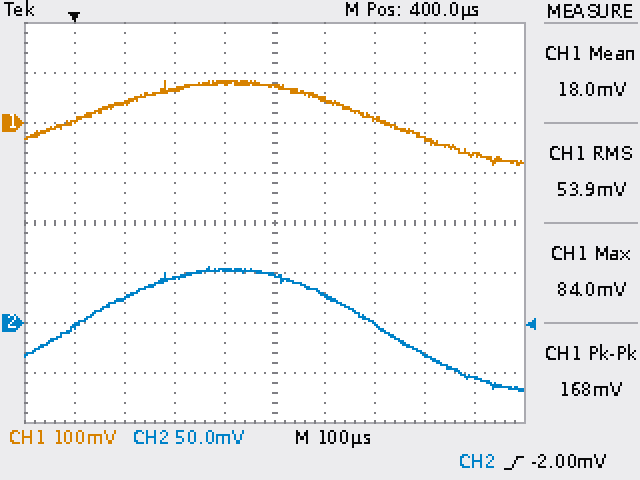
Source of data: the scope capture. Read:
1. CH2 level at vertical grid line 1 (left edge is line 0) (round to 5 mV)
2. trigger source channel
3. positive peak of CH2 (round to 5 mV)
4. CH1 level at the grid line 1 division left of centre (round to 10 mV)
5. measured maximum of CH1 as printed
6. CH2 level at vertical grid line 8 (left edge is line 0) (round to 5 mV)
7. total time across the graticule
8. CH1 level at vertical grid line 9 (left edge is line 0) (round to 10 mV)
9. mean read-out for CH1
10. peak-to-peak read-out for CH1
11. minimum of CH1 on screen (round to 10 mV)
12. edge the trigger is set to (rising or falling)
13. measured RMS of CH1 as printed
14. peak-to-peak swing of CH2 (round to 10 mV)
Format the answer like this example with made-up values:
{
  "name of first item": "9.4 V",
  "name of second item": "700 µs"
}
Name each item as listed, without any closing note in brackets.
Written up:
{
  "CH2 level at vertical grid line 1 (left edge is line 0)": "-5 mV",
  "trigger source channel": "CH2",
  "positive peak of CH2": "55 mV",
  "CH1 level at the grid line 1 division left of centre": "80 mV",
  "measured maximum of CH1 as printed": "84.0 mV",
  "CH2 level at vertical grid line 8 (left edge is line 0)": "-30 mV",
  "total time across the graticule": "1 ms",
  "CH1 level at vertical grid line 9 (left edge is line 0)": "-60 mV",
  "mean read-out for CH1": "18.0 mV",
  "peak-to-peak read-out for CH1": "168 mV",
  "minimum of CH1 on screen": "-80 mV",
  "edge the trigger is set to": "rising",
  "measured RMS of CH1 as printed": "53.9 mV",
  "peak-to-peak swing of CH2": "120 mV"
}
